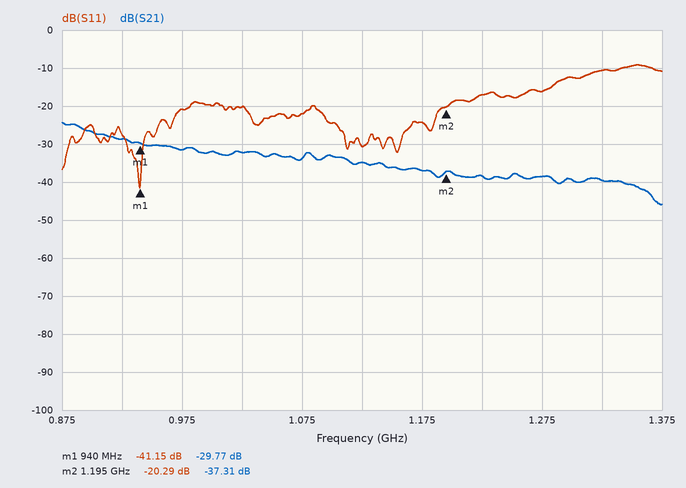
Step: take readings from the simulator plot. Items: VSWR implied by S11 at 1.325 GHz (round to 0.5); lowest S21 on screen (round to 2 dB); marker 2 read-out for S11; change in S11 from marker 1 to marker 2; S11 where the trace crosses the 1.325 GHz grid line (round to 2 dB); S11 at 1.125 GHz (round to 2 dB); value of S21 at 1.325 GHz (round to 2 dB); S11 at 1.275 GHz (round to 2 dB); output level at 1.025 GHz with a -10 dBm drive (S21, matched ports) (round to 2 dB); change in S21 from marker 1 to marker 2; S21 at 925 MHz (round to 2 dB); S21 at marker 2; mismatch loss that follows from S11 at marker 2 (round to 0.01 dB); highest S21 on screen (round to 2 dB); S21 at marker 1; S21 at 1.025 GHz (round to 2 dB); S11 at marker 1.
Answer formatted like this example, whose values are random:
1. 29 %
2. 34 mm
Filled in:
1. 2.0
2. -46 dB
3. -20.29 dB
4. 20.86 dB
5. -10 dB
6. -30 dB
7. -40 dB
8. -16 dB
9. -42 dBm
10. -7.54 dB
11. -28 dB
12. -37.31 dB
13. 0.04 dB
14. -24 dB
15. -29.77 dB
16. -32 dB
17. -41.15 dB
